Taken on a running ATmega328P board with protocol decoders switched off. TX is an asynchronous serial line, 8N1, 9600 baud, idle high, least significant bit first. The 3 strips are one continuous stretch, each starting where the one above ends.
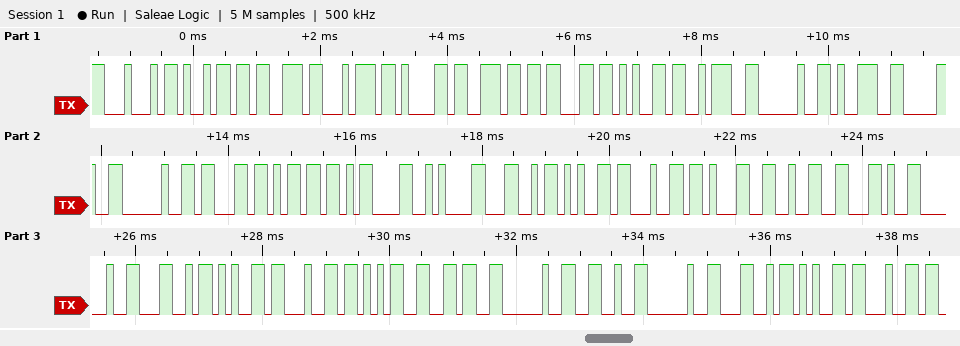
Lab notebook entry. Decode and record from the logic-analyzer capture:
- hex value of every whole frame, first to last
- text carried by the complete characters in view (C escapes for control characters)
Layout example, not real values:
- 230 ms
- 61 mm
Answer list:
- 44 69 73 74 61 6E 63 65 3A 20 39 30 20 63 6D 0D 0A 4C 65 64 31 32 2C 20 4C 65 64 35 36 20 26 20 4C 65 64
- "Distance: 90 cm\r\nLed12, Led56 & Led"
